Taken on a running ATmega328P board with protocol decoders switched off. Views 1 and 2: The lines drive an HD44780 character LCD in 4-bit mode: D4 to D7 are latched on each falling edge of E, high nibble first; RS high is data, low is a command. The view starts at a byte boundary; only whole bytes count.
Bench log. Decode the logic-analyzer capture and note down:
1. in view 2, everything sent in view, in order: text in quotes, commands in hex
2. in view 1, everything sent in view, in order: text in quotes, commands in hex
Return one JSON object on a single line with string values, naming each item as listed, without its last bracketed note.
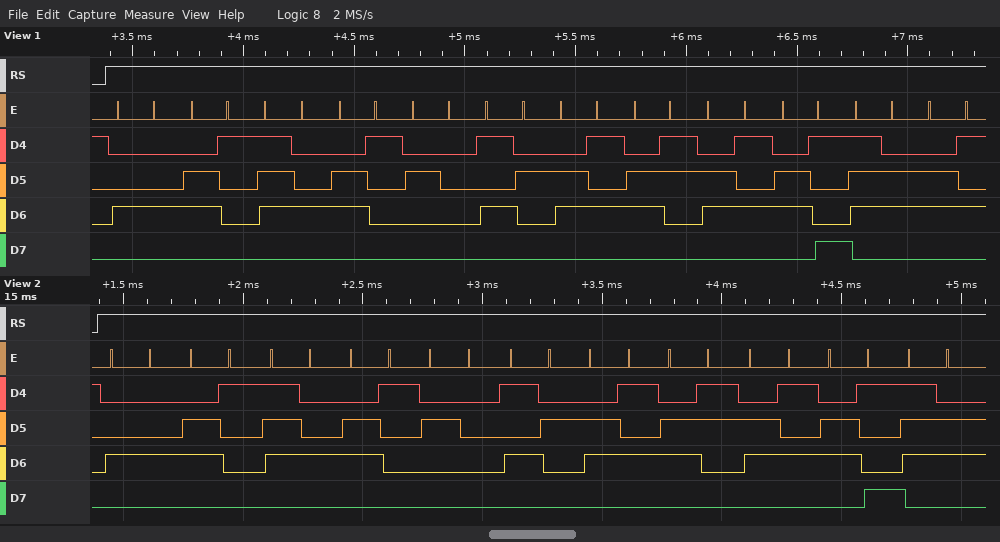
{"in view 2, everything sent in view, in order: text in quotes, commands in hex": "\"Data Receiv\"", "in view 1, everything sent in view, in order: text in quotes, commands in hex": "\"Data Receive\""}
